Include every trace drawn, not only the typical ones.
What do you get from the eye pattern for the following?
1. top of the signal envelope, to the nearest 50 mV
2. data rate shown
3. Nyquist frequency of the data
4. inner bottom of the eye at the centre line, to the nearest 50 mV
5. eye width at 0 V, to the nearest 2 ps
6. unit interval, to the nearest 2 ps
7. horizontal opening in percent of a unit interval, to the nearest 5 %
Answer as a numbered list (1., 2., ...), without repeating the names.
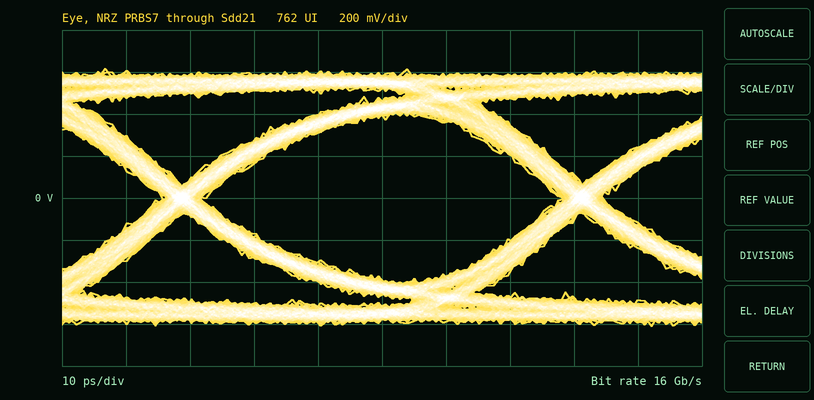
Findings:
1. 600 mV
2. 16 Gb/s
3. 8 GHz
4. -400 mV
5. 56 ps
6. 62 ps
7. 90 %
